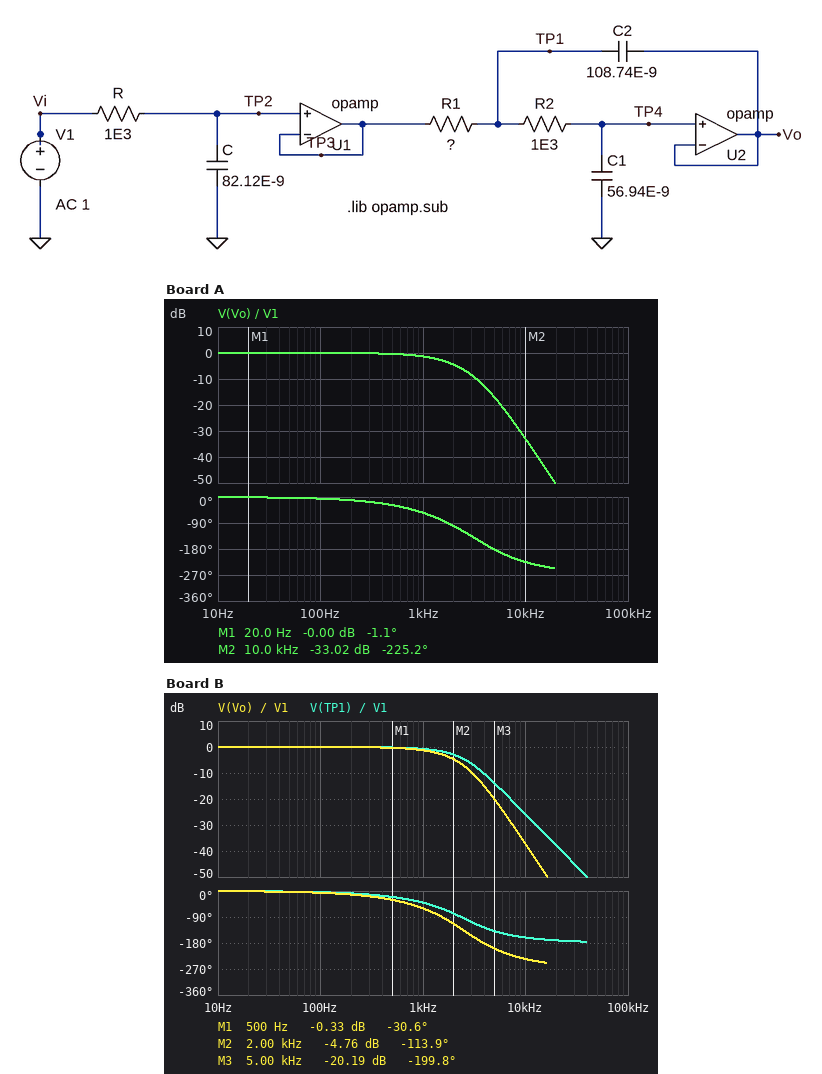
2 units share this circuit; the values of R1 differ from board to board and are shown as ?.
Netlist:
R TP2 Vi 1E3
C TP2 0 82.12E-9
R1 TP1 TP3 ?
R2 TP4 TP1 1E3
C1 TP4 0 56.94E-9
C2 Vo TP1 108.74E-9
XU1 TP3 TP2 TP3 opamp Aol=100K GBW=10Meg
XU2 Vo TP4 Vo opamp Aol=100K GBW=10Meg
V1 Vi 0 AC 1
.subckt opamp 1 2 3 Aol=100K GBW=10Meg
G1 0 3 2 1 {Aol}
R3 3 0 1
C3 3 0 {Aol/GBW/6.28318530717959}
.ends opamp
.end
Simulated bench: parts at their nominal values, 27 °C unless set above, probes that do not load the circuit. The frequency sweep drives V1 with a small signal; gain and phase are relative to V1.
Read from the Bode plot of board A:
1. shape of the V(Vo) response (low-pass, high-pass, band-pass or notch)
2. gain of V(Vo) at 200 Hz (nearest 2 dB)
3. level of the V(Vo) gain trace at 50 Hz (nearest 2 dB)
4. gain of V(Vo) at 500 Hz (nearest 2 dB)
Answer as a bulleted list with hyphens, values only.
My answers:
- low-pass
- 0 dB
- 0 dB
- 0 dB
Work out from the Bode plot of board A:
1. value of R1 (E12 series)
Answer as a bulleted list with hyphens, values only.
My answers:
- 330 Ω
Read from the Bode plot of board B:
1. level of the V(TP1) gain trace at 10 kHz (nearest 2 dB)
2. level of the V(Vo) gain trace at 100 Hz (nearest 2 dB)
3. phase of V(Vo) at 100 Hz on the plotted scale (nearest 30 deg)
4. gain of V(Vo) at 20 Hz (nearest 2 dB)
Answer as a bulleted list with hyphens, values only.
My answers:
- -26 dB
- 0 dB
- 0 deg
- 0 dB
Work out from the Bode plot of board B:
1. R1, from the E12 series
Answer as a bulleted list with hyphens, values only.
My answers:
- 560 Ω
